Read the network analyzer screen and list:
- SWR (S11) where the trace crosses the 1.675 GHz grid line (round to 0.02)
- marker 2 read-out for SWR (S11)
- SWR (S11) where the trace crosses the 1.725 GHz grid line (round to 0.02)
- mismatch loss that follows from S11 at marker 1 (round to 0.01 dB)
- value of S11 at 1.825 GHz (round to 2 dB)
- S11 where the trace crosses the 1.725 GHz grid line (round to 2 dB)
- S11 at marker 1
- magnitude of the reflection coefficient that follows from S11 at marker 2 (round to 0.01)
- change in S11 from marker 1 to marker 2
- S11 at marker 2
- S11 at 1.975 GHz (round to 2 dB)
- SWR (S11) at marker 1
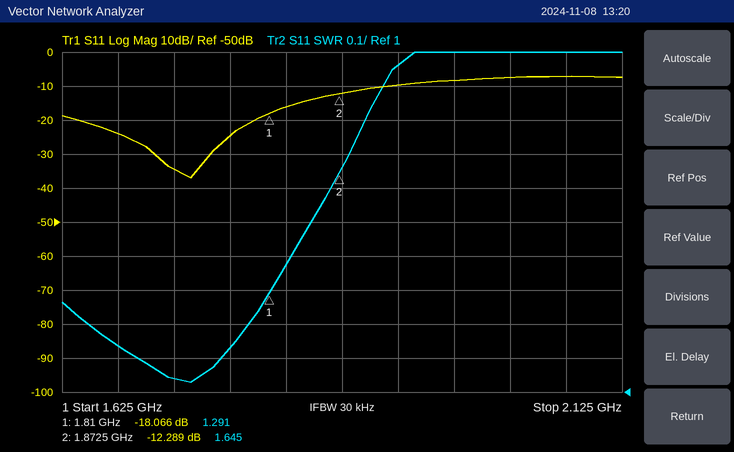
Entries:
1.14
1.645
1.04
0.07 dB
-16 dB
-34 dB
-18.066 dB
0.24
5.777 dB
-12.289 dB
-8 dB
1.291
